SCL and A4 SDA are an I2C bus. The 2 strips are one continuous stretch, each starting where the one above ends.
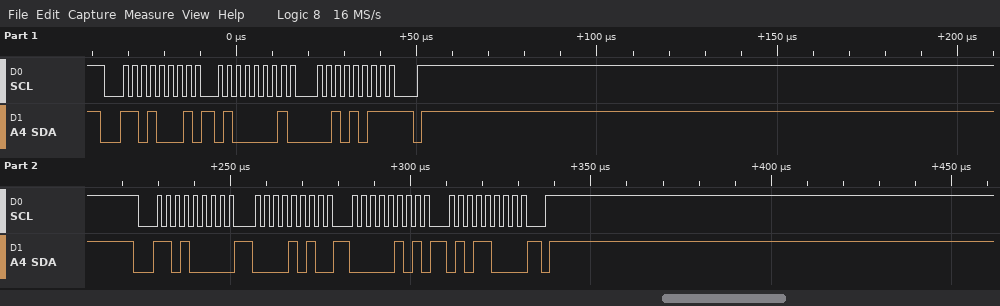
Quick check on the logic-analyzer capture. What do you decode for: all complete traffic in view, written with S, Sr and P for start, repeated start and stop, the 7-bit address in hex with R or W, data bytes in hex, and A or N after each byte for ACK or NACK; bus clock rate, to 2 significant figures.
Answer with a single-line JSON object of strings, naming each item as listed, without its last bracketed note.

{"all complete traffic in view, written with S, Sr and P for start, repeated start and stop, the 7-bit address in hex with R or W, data bytes in hex, and A or N after each byte for ACK or NACK": "S 68R A 41 A 2B N P S 68W A 0A A 05 A 58 A P", "bus clock rate, to 2 significant figures": "400 kHz"}
